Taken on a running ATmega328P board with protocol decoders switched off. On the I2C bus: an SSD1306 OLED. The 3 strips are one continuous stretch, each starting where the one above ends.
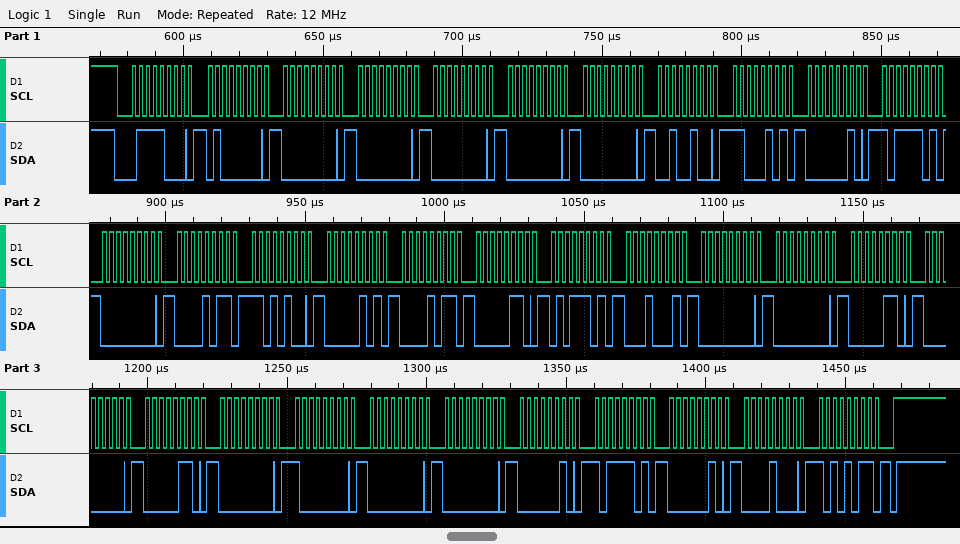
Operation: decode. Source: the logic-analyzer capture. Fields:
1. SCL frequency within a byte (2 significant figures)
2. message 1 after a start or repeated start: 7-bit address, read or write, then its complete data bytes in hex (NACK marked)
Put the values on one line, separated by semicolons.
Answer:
400 kHz; 0x3C write: 40 00 00 00 00 00 24 C5 02 BD 00 0B D4 05 0B 06 5D 11 00 00 06 00 06 00 80 00 00 02 BD 02 08 AB
